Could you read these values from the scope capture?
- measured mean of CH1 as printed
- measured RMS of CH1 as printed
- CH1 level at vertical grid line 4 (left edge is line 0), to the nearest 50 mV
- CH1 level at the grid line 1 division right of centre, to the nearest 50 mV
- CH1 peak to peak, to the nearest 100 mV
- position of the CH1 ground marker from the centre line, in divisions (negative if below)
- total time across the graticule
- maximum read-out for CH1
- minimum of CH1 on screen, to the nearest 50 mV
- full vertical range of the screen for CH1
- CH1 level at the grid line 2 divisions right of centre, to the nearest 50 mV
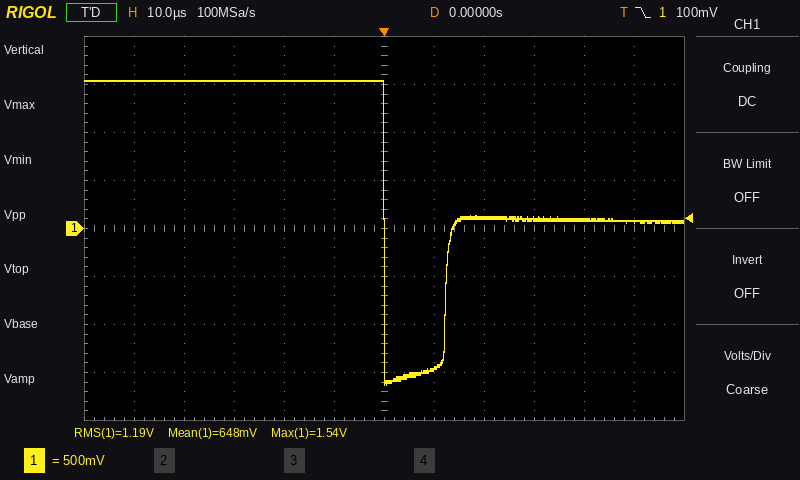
648 mV
1.19 V
1.55 V
-1.45 V
3.20 V
0.0 div
120 µs
1.54 V
-1.60 V
4 V
100 mV
